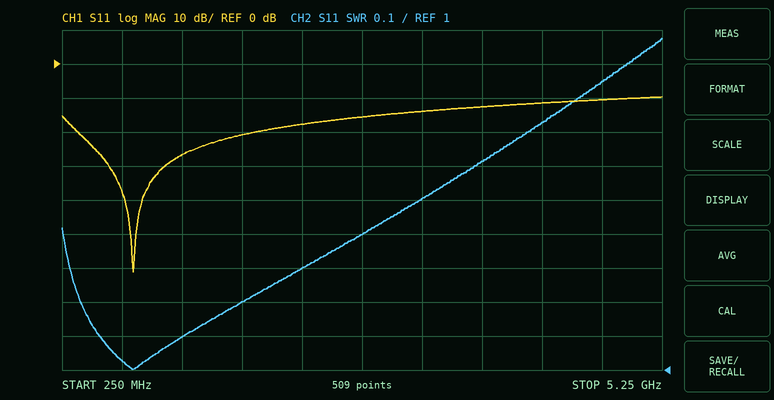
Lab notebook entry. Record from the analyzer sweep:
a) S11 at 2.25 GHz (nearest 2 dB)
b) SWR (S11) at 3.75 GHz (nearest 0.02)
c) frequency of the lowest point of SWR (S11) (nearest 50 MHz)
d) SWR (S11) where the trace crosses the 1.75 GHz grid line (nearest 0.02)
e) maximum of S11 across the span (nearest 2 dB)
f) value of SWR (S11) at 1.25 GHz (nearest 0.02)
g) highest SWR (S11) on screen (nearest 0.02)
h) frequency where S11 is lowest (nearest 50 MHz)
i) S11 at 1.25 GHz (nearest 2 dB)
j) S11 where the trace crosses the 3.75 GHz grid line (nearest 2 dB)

-18 dB
1.62
850 MHz
1.20
-10 dB
1.10
1.98
850 MHz
-26 dB
-12 dB
